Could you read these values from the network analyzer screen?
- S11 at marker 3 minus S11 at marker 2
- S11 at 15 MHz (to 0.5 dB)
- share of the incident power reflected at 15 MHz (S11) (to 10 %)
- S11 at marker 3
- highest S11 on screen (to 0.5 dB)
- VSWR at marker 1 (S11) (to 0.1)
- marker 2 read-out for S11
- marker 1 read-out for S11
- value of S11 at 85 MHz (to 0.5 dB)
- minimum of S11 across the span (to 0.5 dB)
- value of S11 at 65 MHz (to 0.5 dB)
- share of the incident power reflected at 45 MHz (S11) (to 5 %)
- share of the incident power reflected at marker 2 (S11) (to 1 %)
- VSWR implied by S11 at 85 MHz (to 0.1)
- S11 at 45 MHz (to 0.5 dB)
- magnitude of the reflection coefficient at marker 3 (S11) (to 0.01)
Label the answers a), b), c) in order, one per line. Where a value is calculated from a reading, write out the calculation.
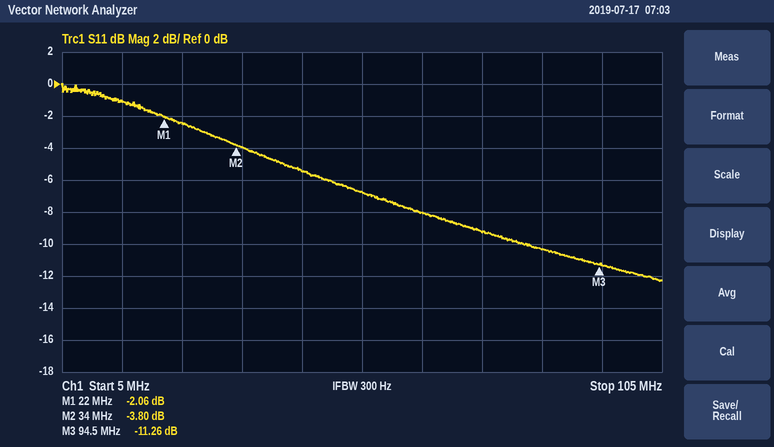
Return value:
a) -11.26 − (-3.8) = -7.46 dB
b) -1.0 dB
c) 10^(-1/10) ≈ 79.4 %, so 80 % to the nearest 10 %
d) -11.26 dB
e) 0.0 dB
f) (1 + 0.7889)/(1 − 0.7889) ≈ 8.5
g) -3.80 dB
h) -2.06 dB
i) -10.5 dB
j) -12.5 dB
k) -8.0 dB
l) 10^(-5.5/10) ≈ 28.2 %, so 30 % to the nearest 5 %
m) 10^(-3.8/10) ≈ 42 %
n) |Γ| = 10^(-10.5/20) = 0.2985; VSWR = (1 + 0.2985)/(1 − 0.2985) ≈ 1.9
o) -5.5 dB
p) 10^(-11.26/20) ≈ 0.27
